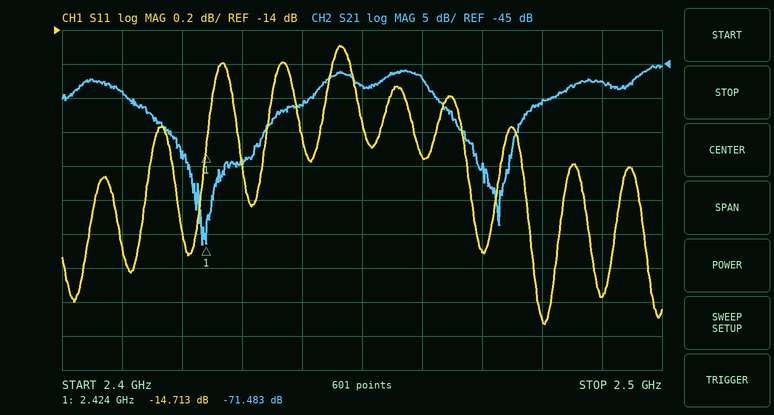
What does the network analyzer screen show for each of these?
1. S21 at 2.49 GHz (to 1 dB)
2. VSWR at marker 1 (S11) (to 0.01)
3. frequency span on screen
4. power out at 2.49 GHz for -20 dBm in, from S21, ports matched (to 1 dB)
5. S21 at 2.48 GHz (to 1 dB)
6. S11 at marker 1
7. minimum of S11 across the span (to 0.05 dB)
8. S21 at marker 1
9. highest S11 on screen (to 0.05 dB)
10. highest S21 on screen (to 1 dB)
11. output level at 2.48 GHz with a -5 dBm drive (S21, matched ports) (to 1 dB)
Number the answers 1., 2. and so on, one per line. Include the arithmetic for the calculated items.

1. -48 dB
2. (1 + 0.1838)/(1 − 0.1838) ≈ 1.45
3. 100 MHz
4. -20 dBm + (-48 dB) = -68 dBm
5. -51 dB
6. -14.713 dB
7. -15.75 dB
8. -71.483 dB
9. -14.10 dB
10. -45 dB
11. -5 dBm + (-51 dB) = -56 dBm
